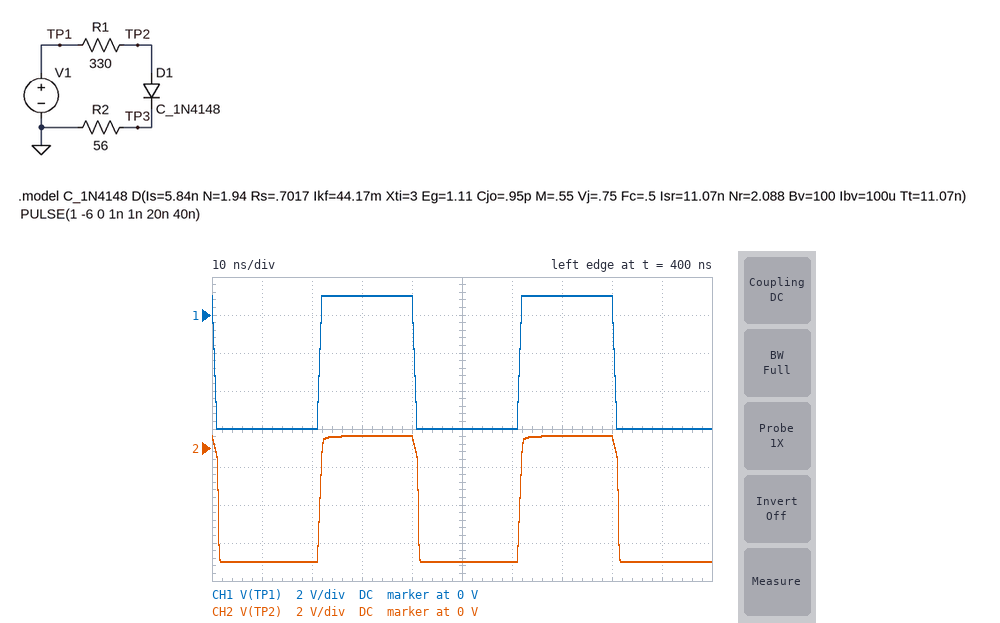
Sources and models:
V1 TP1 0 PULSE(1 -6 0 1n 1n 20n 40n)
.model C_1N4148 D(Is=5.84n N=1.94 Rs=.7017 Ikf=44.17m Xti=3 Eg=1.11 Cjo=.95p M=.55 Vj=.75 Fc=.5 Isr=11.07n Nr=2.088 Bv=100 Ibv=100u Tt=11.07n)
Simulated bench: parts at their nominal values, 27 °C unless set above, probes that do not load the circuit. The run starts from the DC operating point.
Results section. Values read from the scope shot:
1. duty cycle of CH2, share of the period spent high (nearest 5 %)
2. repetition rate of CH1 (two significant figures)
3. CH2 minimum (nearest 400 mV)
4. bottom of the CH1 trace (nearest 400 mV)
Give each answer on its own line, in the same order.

50 %
25 MHz
-6.0 V
-6.0 V
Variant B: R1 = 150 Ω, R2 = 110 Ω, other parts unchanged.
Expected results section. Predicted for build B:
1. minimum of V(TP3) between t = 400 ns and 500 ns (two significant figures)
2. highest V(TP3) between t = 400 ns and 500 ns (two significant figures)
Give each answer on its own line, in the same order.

-2.7 V
480 mV
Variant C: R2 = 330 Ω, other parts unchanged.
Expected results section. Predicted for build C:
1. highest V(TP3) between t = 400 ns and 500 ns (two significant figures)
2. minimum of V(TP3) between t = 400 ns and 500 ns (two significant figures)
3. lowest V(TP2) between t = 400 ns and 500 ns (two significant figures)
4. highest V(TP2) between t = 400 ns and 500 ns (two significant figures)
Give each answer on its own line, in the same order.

1.0 V
-3.2 V
-6.0 V
780 mV
